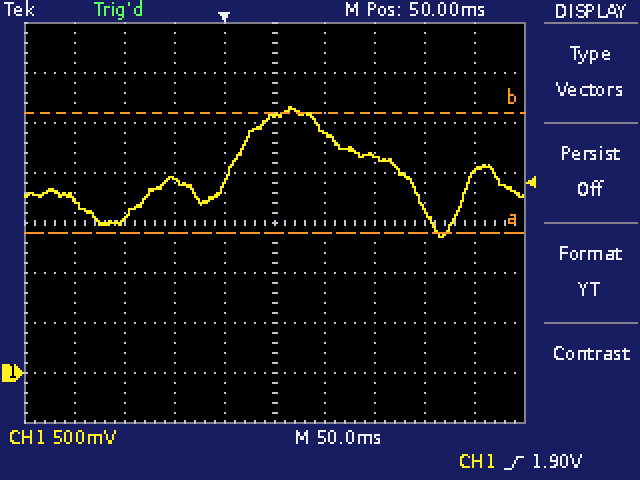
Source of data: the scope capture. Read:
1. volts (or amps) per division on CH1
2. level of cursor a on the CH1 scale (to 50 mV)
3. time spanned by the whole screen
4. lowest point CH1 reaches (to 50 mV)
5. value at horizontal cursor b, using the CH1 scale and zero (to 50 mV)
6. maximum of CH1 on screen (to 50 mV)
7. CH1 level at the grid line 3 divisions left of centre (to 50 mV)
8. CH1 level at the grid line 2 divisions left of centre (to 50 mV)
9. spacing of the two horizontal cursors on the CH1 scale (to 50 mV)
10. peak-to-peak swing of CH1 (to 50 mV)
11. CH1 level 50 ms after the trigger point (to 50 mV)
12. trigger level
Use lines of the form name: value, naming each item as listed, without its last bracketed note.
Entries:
volts (or amps) per division on CH1: 500 mV
level of cursor a on the CH1 scale: 1.40 V
time spanned by the whole screen: 500 ms
lowest point CH1 reaches: 1.35 V
value at horizontal cursor b, using the CH1 scale and zero: 2.60 V
maximum of CH1 on screen: 2.65 V
CH1 level at the grid line 3 divisions left of centre: 1.55 V
CH1 level at the grid line 2 divisions left of centre: 1.95 V
spacing of the two horizontal cursors on the CH1 scale: 1.20 V
peak-to-peak swing of CH1: 1.30 V
CH1 level 50 ms after the trigger point: 2.60 V
trigger level: 1.90 V
